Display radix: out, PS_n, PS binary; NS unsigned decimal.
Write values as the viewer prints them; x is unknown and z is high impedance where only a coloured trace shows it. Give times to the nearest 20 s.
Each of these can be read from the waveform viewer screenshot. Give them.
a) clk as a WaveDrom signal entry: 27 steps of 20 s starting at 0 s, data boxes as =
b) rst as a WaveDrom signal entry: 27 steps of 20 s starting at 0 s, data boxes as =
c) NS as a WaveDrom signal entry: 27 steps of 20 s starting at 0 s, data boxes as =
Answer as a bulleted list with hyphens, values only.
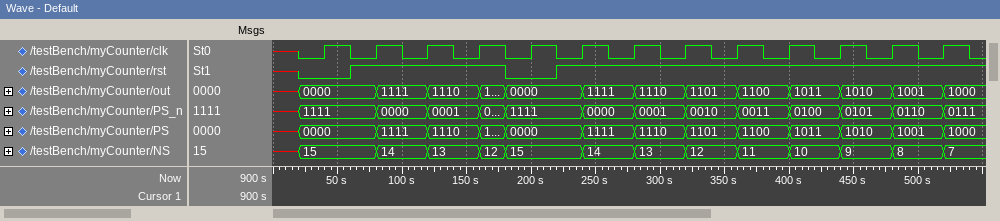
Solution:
- {name: 'clk', wave: 'x01010101010101010101010101'}
- {name: 'rst', wave: 'x0.1.....0.1...............'}
- {name: 'NS', wave: 'x=..=.=.==..=.=.=.=.=.=.=.=', data: '15 14 13 12 15 14 13 12 11 10 9 8 7'}
